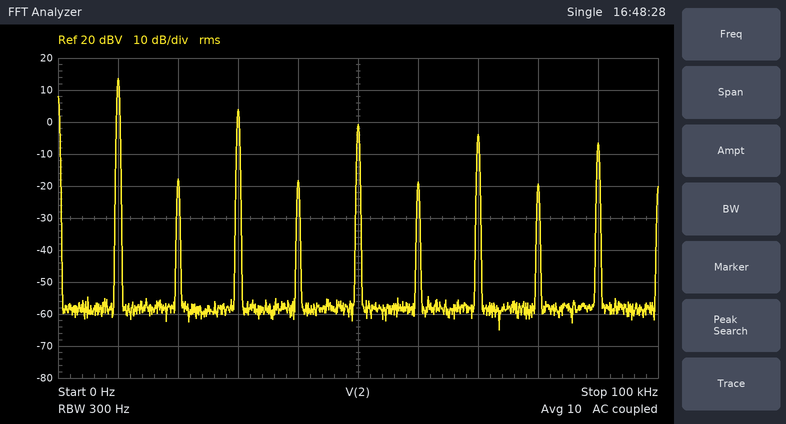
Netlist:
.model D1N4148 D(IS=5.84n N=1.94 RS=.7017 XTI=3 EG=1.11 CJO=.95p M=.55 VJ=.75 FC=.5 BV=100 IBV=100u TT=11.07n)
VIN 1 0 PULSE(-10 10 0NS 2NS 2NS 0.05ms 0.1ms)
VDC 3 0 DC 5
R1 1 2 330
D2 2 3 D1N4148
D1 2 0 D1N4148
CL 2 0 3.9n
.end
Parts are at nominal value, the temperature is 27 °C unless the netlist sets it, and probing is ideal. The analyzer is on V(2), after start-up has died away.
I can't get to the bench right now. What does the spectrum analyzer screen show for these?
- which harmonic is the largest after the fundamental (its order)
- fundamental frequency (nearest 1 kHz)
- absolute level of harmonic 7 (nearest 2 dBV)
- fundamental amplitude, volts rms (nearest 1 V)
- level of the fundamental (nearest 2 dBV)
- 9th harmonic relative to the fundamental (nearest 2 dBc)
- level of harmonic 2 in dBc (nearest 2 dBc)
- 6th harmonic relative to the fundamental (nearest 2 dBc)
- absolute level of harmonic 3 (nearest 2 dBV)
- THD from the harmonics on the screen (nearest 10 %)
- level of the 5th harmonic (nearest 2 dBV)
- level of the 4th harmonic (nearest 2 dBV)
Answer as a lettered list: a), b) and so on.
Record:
a) 3
b) 10 kHz
c) -4 dBV
d) 5 V
e) 14 dBV
f) -20 dBc
g) -32 dBc
h) -32 dBc
i) 4 dBV
j) 40 %
k) 0 dBV
l) -18 dBV
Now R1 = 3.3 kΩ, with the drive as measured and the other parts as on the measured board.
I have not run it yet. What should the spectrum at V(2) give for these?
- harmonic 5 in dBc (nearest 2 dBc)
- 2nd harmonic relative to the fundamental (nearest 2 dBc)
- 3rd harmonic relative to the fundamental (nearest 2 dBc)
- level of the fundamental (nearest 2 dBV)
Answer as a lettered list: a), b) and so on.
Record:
a) -20 dBc
b) -16 dBc
c) -12 dBc
d) 12 dBV
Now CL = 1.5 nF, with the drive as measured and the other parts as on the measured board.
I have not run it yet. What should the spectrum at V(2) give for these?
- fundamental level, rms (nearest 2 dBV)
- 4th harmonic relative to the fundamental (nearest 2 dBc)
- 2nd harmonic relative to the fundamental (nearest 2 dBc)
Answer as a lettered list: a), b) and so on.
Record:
a) 14 dBV
b) -40 dBc
c) -40 dBc
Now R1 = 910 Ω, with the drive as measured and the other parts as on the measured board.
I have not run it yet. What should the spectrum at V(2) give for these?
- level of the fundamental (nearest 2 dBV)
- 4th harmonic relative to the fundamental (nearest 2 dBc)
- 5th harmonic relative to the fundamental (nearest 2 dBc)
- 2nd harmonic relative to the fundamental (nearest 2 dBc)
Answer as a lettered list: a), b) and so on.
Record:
a) 14 dBV
b) -26 dBc
c) -16 dBc
d) -24 dBc
